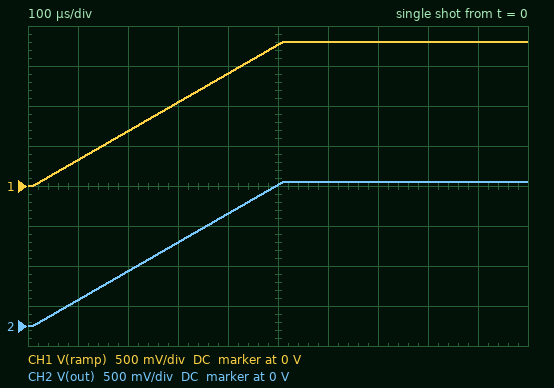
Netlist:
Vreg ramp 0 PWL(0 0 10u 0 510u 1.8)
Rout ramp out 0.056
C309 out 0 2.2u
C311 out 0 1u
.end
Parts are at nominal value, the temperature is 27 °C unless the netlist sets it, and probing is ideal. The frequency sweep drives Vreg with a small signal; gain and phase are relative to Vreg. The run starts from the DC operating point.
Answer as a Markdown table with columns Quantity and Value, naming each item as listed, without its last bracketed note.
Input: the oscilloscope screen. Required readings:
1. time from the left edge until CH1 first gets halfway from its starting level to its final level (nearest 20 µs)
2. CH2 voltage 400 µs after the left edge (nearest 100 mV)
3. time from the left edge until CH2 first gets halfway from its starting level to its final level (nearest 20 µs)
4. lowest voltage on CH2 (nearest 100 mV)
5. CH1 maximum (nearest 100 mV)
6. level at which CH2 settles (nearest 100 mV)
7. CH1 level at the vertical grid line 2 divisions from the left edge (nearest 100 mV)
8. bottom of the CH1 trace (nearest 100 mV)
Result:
| Quantity | Value |
|---|---|
| time from the left edge until CH1 first gets halfway from its starting level to its final level | 260 µs |
| CH2 voltage 400 µs after the left edge | 1.4 V |
| time from the left edge until CH2 first gets halfway from its starting level to its final level | 260 µs |
| lowest voltage on CH2 | 0 V |
| CH1 maximum | 1.8 V |
| level at which CH2 settles | 1.8 V |
| CH1 level at the vertical grid line 2 divisions from the left edge | 700 mV |
| bottom of the CH1 trace | 0 V |
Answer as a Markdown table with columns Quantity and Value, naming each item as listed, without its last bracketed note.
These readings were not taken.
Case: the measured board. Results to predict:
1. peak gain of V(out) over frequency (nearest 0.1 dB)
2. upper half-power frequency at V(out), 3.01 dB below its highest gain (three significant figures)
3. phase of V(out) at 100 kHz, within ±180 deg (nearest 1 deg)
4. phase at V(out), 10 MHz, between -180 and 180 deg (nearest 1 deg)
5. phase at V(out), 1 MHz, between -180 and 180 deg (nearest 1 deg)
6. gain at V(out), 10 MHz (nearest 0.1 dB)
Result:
| Quantity | Value |
|---|---|
| peak gain of V(out) over frequency | 0 dB |
| upper half-power frequency at V(out), 3.01 dB below its highest gain | 888 kHz |
| phase of V(out) at 100 kHz, within ±180 deg | -6 deg |
| phase at V(out), 10 MHz, between -180 and 180 deg | -85 deg |
| phase at V(out), 1 MHz, between -180 and 180 deg | -48 deg |
| gain at V(out), 10 MHz | -21.1 dB |
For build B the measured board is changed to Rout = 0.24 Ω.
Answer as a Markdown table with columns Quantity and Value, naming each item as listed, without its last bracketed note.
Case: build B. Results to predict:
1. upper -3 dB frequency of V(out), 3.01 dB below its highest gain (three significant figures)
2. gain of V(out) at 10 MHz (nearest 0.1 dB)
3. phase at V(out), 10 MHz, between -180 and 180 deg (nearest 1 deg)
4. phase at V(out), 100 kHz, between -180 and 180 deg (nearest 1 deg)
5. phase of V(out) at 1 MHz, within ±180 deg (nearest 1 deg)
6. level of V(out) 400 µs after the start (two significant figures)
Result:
| Quantity | Value |
|---|---|
| upper -3 dB frequency of V(out), 3.01 dB below its highest gain | 207 kHz |
| gain of V(out) at 10 MHz | -33.7 dB |
| phase at V(out), 10 MHz, between -180 and 180 deg | -89 deg |
| phase at V(out), 100 kHz, between -180 and 180 deg | -26 deg |
| phase of V(out) at 1 MHz, within ±180 deg | -78 deg |
| level of V(out) 400 µs after the start | 1.4 V |
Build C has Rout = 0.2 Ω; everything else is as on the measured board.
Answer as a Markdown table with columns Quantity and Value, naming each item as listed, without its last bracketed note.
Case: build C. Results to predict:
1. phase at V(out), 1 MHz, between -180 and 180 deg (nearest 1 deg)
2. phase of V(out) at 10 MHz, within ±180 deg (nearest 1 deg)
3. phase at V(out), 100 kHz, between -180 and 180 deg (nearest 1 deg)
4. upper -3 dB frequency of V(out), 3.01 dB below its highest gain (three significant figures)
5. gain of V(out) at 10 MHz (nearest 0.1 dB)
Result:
| Quantity | Value |
|---|---|
| phase at V(out), 1 MHz, between -180 and 180 deg | -76 deg |
| phase of V(out) at 10 MHz, within ±180 deg | -89 deg |
| phase at V(out), 100 kHz, between -180 and 180 deg | -22 deg |
| upper -3 dB frequency of V(out), 3.01 dB below its highest gain | 249 kHz |
| gain of V(out) at 10 MHz | -32.1 dB |
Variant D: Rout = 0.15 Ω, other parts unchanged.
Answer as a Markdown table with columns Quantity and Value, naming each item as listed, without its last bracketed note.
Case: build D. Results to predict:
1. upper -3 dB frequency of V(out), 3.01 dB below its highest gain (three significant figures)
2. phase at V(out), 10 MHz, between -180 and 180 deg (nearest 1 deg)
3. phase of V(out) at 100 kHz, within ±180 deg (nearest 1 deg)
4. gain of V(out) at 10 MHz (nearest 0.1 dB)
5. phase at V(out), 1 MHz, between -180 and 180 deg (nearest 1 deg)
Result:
| Quantity | Value |
|---|---|
| upper -3 dB frequency of V(out), 3.01 dB below its highest gain | 332 kHz |
| phase at V(out), 10 MHz, between -180 and 180 deg | -88 deg |
| phase of V(out) at 100 kHz, within ±180 deg | -17 deg |
| gain of V(out) at 10 MHz | -29.6 dB |
| phase at V(out), 1 MHz, between -180 and 180 deg | -72 deg |
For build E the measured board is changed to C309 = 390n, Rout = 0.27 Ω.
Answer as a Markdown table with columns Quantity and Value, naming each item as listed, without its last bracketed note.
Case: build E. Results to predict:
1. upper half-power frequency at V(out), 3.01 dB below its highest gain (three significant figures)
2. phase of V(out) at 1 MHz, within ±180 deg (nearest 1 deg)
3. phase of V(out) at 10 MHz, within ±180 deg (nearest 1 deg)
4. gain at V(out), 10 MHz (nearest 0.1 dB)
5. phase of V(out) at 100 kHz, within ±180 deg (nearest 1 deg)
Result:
| Quantity | Value |
|---|---|
| upper half-power frequency at V(out), 3.01 dB below its highest gain | 424 kHz |
| phase of V(out) at 1 MHz, within ±180 deg | -67 deg |
| phase of V(out) at 10 MHz, within ±180 deg | -88 deg |
| gain at V(out), 10 MHz | -27.5 dB |
| phase of V(out) at 100 kHz, within ±180 deg | -13 deg |
